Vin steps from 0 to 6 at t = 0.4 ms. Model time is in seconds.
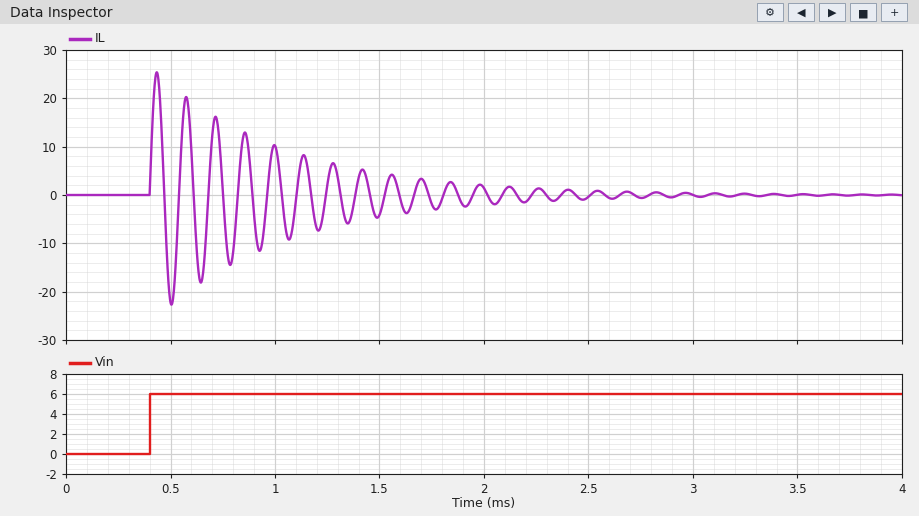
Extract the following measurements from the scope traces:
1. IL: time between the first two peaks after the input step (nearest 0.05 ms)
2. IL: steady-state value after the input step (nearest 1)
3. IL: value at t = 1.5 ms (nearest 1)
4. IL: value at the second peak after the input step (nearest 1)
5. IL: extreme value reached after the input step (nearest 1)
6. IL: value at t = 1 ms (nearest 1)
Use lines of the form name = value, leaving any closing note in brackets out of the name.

IL: time between the first two peaks after the input step = 0.15 ms
IL: steady-state value after the input step = 0
IL: value at t = 1.5 ms = -4
IL: value at the second peak after the input step = 20
IL: extreme value reached after the input step = 25
IL: value at t = 1 ms = 10
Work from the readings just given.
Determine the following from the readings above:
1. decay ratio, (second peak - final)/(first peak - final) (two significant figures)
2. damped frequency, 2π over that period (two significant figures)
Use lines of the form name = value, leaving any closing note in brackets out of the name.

decay ratio, (second peak - final)/(first peak - final) = 0.80
damped frequency, 2π over that period = 42 rad/ms
